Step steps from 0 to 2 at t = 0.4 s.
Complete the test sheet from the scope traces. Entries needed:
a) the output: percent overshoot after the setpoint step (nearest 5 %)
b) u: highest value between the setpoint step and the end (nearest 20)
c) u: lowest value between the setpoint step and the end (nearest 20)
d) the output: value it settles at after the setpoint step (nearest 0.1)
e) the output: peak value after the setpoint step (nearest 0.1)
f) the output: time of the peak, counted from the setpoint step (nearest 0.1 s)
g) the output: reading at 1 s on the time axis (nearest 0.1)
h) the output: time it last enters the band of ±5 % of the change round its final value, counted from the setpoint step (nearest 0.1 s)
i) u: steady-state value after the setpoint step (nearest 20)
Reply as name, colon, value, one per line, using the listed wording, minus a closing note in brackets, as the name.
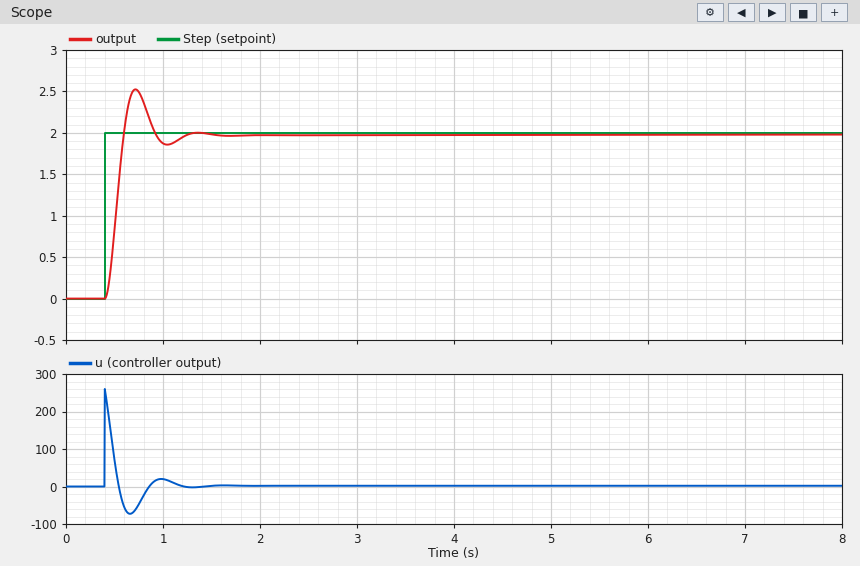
the output: percent overshoot after the setpoint step: 25 %
u: highest value between the setpoint step and the end: 260
u: lowest value between the setpoint step and the end: -80
the output: value it settles at after the setpoint step: 2.0
the output: peak value after the setpoint step: 2.5
the output: time of the peak, counted from the setpoint step: 0.3 s
the output: reading at 1 s on the time axis: 1.9
the output: time it last enters the band of ±5 % of the change round its final value, counted from the setpoint step: 0.7 s
u: steady-state value after the setpoint step: 0
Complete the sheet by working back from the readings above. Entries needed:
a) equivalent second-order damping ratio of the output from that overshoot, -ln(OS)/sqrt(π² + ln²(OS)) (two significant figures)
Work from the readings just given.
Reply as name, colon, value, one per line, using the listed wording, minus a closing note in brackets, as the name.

equivalent second-order damping ratio of the output from that overshoot, -ln(OS)/sqrt(π² + ln²(OS)): 0.40
